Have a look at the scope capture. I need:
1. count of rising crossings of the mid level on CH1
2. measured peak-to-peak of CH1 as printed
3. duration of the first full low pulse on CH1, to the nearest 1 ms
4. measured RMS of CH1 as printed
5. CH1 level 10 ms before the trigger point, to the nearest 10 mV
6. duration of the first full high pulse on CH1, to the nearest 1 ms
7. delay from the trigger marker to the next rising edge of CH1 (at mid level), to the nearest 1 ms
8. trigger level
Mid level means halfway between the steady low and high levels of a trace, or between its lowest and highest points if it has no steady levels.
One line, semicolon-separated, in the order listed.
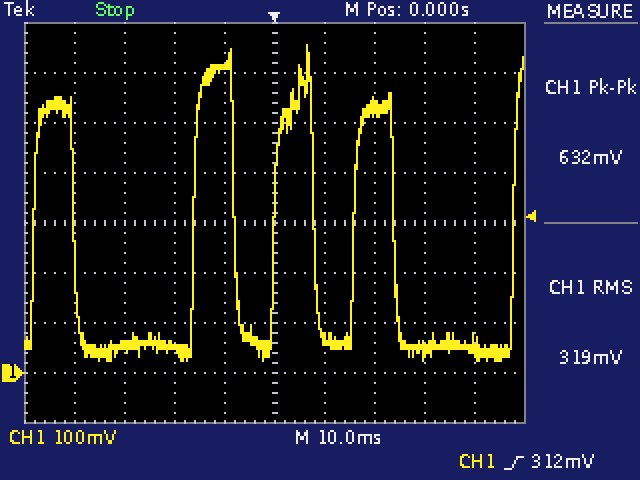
5; 632 mV; 24 ms; 319 mV; 620 mV; 8 ms; 16 ms; 312 mV
